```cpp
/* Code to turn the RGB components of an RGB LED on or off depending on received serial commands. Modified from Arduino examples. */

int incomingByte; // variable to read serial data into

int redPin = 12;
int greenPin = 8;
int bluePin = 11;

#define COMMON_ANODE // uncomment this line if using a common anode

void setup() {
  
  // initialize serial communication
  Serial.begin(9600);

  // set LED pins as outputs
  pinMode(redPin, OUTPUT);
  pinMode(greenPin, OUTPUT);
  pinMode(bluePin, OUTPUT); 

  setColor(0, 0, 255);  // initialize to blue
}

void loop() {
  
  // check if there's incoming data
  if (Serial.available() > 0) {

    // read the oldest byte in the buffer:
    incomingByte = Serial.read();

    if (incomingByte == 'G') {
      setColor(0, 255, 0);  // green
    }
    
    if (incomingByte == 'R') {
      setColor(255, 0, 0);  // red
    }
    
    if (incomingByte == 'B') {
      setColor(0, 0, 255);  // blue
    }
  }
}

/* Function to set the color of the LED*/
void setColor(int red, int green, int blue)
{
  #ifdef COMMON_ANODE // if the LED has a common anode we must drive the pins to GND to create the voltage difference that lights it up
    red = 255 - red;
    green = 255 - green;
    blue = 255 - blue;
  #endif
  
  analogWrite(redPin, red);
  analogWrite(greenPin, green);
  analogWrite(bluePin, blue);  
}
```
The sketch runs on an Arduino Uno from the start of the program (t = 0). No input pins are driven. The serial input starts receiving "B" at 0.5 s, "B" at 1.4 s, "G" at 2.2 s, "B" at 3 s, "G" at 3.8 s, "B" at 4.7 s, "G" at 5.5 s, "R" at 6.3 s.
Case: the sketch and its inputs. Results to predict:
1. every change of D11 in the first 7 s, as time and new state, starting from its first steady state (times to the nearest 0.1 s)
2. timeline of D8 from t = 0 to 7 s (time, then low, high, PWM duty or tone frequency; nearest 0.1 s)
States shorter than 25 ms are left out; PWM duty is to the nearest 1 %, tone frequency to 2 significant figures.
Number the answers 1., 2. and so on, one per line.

1. 0 s low; 2.2 s high; 3 s low; 3.8 s high; 4.7 s low; 5.5 s high
2. 0 s high; 2.2 s low; 3 s high; 3.8 s low; 4.7 s high; 5.5 s low; 6.3 s high
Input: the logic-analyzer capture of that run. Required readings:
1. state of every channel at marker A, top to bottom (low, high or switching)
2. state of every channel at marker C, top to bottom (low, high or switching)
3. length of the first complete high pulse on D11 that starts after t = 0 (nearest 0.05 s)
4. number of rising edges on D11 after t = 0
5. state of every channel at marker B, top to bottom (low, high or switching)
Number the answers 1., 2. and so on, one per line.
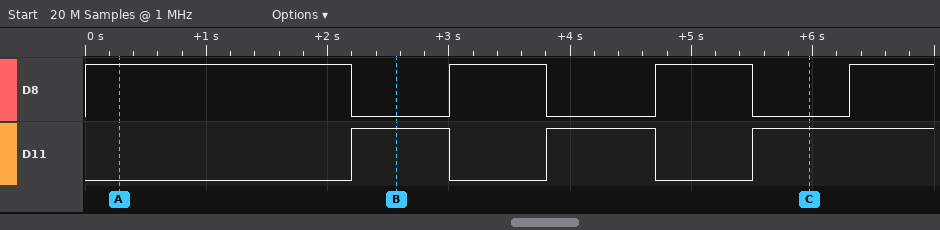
1. D8 high, D11 low
2. D8 low, D11 high
3. 0.80 s
4. 3
5. D8 low, D11 high
